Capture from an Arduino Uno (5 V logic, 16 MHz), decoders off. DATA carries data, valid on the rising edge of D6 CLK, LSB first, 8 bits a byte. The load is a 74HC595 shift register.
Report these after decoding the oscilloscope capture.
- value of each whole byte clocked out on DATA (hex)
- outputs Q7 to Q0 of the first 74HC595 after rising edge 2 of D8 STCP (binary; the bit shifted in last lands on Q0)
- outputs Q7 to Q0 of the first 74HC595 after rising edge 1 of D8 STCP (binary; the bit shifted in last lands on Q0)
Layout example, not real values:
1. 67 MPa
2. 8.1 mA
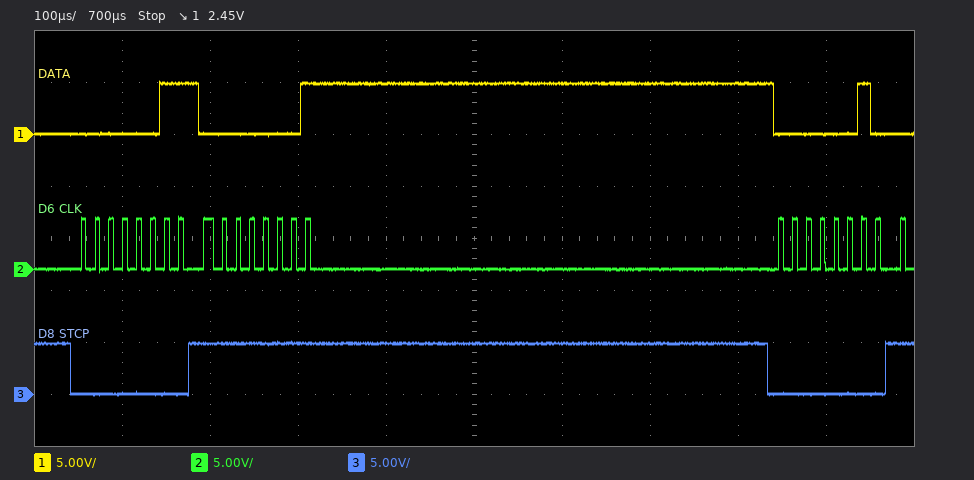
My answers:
1. C0 80 40
2. 00000010
3. 00000011
